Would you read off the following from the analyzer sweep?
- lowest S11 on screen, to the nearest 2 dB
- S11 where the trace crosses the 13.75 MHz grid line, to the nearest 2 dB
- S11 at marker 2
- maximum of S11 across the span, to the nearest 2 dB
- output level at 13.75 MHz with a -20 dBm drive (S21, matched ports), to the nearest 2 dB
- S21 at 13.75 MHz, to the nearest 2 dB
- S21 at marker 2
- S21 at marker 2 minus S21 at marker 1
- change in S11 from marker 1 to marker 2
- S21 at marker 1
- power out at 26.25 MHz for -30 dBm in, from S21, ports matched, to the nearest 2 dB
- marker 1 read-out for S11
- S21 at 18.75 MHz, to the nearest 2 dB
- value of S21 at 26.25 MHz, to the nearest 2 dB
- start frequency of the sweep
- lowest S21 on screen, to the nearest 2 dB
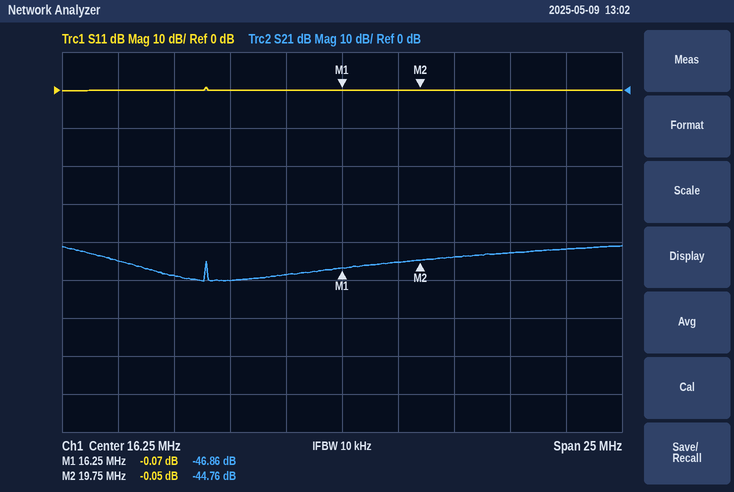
0 dB
0 dB
-0.05 dB
0 dB
-68 dBm
-48 dB
-44.76 dB
2.10 dB
0.02 dB
-46.86 dB
-72 dBm
-0.07 dB
-46 dB
-42 dB
3.75 MHz
-50 dB
